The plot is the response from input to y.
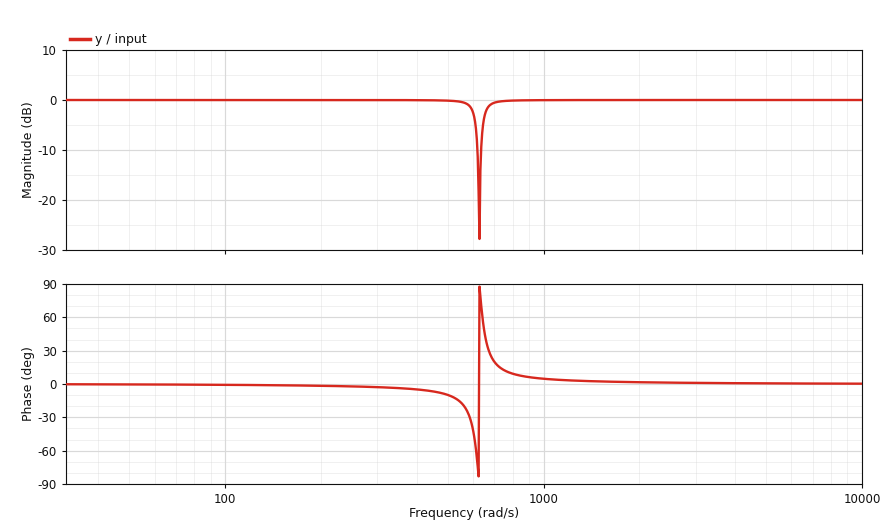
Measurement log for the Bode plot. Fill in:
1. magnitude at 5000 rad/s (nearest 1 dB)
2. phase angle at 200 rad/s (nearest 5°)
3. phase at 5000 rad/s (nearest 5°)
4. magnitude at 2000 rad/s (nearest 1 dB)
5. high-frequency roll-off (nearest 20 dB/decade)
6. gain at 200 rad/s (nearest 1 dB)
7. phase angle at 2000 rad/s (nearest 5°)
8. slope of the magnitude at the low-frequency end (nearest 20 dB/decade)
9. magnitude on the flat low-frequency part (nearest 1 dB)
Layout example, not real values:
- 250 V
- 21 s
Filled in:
- 0 dB
- 0°
- 0°
- 0 dB
- 0 dB/decade
- 0 dB
- 0°
- 0 dB/decade
- 0 dB
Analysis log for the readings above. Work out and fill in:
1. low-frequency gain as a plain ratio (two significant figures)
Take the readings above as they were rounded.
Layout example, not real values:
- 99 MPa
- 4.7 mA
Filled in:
- 1.0
